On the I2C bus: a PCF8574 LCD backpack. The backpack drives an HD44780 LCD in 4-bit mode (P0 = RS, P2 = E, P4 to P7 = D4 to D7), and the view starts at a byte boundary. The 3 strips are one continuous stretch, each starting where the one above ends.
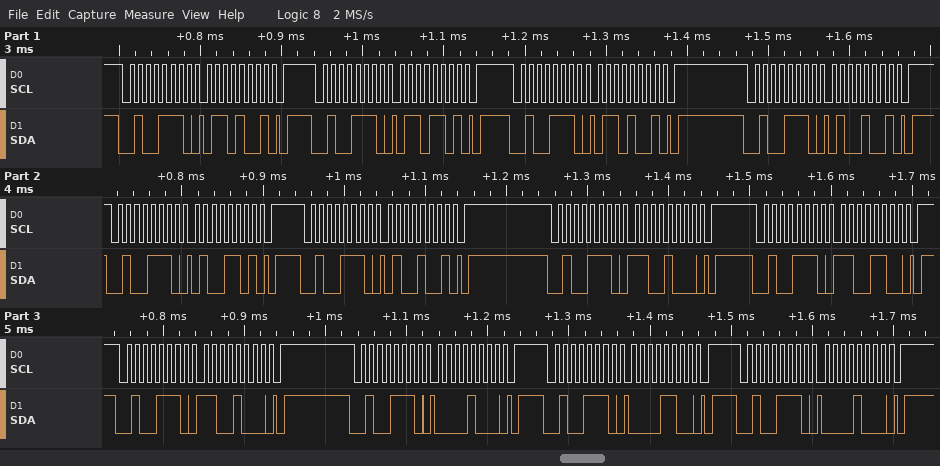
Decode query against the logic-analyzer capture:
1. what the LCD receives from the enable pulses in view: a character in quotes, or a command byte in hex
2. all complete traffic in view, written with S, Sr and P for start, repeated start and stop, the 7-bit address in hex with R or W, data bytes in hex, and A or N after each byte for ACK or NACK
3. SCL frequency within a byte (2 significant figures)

'd' 0xC0
S 27W A 69 A P S 27W A 6D A P S 27W A 69 A P S 27W A 49 A P S 27W A 4D A P S 27W A 49 A P S 27W A C8 A P S 27W A CC A P S 27W A C8 A P S 27W A 08 A P S 27W A 0C A P S 27W A 08 A P
100 kHz
